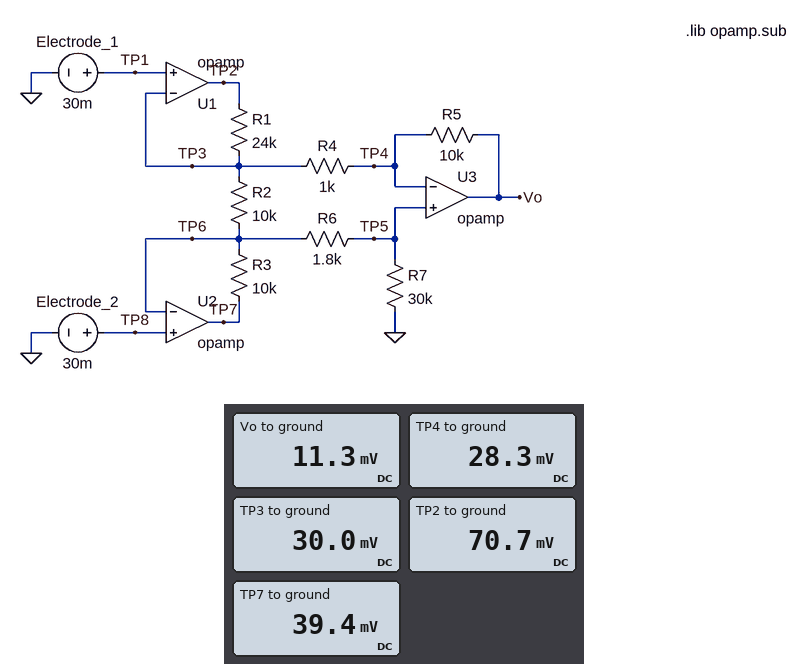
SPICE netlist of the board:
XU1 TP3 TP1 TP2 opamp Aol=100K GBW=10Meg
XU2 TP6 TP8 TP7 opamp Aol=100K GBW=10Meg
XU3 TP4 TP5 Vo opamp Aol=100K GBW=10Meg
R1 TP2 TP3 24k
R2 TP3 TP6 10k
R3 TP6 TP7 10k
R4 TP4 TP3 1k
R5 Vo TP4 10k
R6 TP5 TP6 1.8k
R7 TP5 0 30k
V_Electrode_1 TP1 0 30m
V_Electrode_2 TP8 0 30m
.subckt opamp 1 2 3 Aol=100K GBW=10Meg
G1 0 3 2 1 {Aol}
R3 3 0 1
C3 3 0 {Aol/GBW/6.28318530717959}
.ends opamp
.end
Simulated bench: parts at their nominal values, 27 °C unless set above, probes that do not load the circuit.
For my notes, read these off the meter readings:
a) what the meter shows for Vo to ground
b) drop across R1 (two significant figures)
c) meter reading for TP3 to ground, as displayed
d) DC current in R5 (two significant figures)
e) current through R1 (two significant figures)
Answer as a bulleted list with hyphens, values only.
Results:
- 11.3 mV
- 41 mV
- 30.0 mV
- 1.7 µA
- 1.7 µA
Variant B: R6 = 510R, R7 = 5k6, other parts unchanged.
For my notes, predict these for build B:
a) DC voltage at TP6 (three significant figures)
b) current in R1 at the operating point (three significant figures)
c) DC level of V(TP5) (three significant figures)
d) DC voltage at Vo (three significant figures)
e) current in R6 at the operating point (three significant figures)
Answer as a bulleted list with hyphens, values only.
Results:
- 30.0 mV
- 2.50 µA
- 27.5 mV
- 2.46 mV
- 4.91 µA
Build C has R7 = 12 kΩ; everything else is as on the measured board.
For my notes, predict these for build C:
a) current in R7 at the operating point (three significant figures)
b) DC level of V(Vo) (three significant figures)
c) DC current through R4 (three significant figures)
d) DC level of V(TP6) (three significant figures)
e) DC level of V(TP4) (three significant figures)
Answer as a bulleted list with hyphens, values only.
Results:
- 2.17 µA
- -13.0 mV
- 3.91 µA
- 30.0 mV
- 26.1 mV
